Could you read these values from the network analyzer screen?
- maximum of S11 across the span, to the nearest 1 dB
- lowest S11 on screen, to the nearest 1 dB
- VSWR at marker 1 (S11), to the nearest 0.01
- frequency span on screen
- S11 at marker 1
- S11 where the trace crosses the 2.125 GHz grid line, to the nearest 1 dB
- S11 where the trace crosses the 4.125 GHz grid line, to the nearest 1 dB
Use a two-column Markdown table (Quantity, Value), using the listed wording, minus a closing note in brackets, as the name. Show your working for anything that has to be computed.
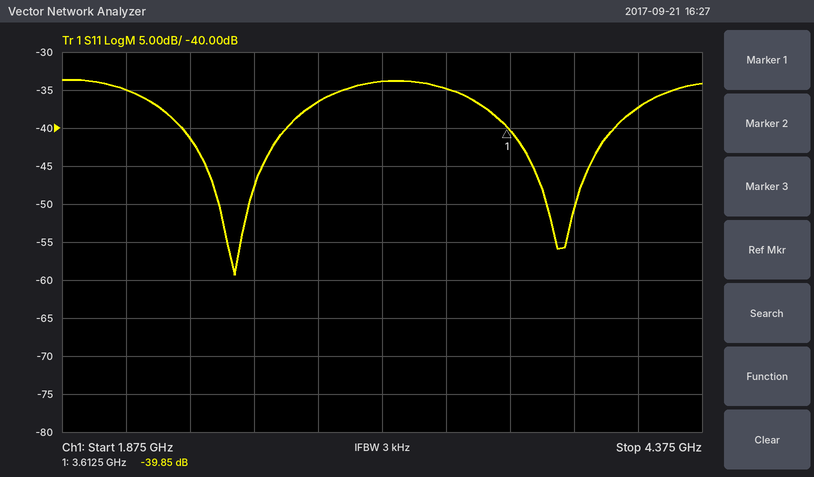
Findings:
| Quantity | Value |
|---|---|
| maximum of S11 across the span, to the nearest 1 dB | -34 dB |
| lowest S11 on screen, to the nearest 1 dB | -59 dB |
| VSWR at marker 1 (S11), to the nearest 0.01 | (1 + 0.0102)/(1 − 0.0102) ≈ 1.02 |
| frequency span on screen | 2.5 GHz |
| S11 at marker 1 | -39.85 dB |
| S11 where the trace crosses the 2.125 GHz grid line, to the nearest 1 dB | -35 dB |
| S11 where the trace crosses the 4.125 GHz grid line, to the nearest 1 dB | -37 dB |
